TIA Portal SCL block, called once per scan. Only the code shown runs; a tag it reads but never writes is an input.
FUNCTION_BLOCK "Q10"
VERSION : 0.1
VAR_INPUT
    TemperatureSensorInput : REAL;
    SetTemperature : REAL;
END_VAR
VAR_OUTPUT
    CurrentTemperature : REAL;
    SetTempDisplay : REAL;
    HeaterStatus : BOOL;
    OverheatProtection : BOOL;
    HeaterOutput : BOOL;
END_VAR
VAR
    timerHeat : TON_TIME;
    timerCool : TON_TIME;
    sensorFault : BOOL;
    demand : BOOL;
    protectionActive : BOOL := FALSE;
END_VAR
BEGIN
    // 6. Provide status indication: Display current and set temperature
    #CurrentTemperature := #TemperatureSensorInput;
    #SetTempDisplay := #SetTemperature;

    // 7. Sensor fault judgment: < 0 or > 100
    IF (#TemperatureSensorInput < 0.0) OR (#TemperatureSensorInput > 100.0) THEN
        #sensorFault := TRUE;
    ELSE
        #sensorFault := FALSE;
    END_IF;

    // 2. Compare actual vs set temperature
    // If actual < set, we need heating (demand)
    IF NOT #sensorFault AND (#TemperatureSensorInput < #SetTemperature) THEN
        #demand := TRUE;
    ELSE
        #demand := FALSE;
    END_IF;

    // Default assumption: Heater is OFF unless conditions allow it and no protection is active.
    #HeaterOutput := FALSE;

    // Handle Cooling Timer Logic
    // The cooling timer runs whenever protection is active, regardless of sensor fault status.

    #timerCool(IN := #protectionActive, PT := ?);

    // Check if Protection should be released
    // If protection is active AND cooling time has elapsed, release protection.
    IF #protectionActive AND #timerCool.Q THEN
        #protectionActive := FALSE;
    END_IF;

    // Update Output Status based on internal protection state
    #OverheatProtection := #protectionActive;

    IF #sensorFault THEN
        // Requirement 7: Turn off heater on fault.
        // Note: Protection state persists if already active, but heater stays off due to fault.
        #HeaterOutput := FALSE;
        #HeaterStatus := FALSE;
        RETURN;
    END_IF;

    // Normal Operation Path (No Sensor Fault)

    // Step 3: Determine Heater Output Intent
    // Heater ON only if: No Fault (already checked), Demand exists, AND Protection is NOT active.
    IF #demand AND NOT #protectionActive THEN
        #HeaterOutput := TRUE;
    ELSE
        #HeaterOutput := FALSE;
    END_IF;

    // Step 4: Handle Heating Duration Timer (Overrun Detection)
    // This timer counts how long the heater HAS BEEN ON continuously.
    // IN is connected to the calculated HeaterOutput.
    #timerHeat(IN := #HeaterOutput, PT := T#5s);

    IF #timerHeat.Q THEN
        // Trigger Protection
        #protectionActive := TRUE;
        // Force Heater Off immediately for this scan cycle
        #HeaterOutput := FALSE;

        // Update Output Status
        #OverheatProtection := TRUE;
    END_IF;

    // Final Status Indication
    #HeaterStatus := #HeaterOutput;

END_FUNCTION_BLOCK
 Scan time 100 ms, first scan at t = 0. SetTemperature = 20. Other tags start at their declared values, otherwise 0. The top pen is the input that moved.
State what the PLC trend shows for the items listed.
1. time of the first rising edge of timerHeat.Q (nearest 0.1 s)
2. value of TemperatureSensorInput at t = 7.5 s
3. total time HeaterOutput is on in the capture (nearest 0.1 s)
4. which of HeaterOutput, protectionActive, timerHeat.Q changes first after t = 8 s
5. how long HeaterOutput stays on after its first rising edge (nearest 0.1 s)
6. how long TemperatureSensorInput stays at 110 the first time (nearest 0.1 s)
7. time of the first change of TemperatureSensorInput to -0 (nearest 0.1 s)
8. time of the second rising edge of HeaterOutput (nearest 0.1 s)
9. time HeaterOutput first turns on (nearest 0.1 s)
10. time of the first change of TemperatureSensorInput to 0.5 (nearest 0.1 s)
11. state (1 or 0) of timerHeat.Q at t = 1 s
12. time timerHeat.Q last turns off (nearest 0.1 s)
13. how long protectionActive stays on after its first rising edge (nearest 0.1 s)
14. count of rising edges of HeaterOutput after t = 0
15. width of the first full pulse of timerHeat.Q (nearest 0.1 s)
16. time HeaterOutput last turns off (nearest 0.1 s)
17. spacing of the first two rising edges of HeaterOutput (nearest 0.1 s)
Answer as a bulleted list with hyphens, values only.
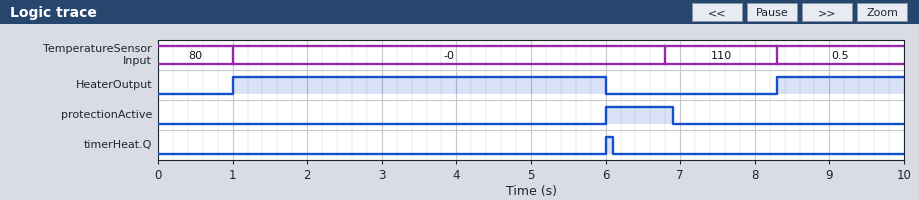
- 6.0 s
- 110
- 6.7 s
- HeaterOutput
- 5.0 s
- 1.5 s
- 1.0 s
- 8.3 s
- 1.0 s
- 8.3 s
- 0
- 6.1 s
- 0.9 s
- 2
- 0.1 s
- 6.0 s
- 7.3 s
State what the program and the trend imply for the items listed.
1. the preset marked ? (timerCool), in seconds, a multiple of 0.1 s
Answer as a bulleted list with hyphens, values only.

- 0.8 s
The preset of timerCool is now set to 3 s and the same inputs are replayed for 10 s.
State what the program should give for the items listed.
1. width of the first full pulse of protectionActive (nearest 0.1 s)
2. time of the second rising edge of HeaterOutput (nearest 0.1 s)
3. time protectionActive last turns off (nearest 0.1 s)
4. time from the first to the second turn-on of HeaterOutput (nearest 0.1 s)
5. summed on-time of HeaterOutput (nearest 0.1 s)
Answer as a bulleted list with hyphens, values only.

- 3.1 s
- 9.1 s
- 9.1 s
- 8.1 s
- 5.9 s
